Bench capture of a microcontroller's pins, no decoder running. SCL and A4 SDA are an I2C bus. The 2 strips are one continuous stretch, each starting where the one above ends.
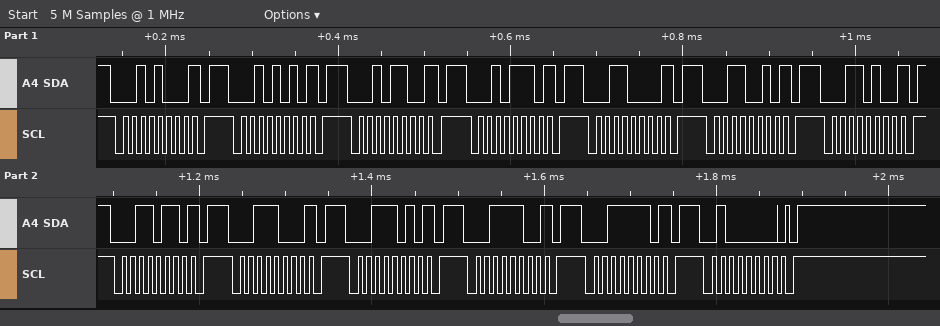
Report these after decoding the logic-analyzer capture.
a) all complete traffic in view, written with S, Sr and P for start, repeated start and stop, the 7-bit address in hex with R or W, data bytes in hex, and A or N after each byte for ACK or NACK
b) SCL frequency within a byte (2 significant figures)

S 14W N P S 15W N P S 16W N P S 17W N P S 18W N P S 19W N P S 1AW N P S 1BW N P S 1CW N P S 1DW N P S 1EW N P S 1FW N P S 20W A P
100 kHz
